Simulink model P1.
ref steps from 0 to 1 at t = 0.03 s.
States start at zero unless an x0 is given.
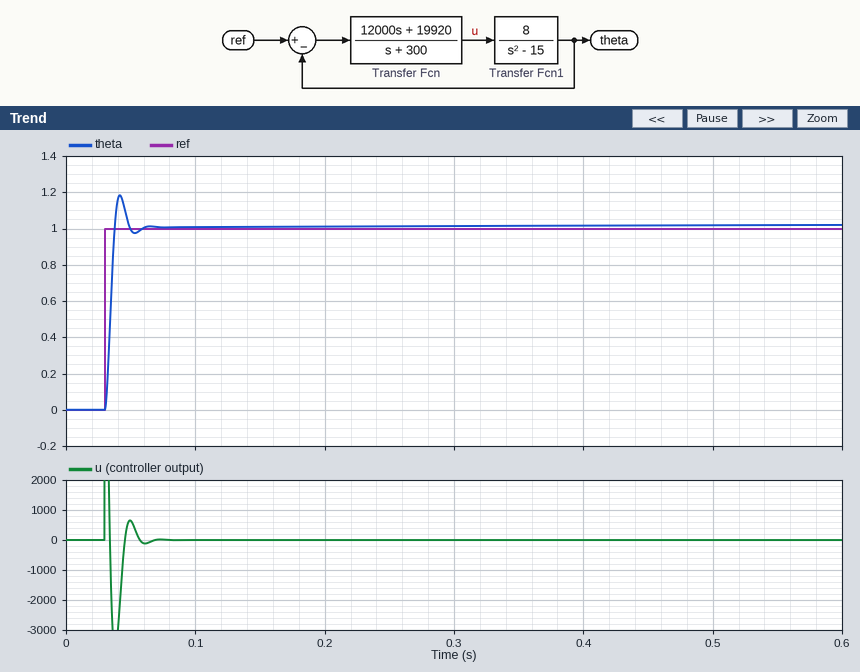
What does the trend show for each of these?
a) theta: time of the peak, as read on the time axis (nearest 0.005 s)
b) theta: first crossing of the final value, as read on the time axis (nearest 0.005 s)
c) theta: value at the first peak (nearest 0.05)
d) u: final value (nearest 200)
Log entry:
0.040 s
0.040 s
1.20
0
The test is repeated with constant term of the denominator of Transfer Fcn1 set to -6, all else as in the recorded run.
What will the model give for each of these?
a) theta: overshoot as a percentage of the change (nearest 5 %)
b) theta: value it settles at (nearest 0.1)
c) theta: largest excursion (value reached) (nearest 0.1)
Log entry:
15 %
1.0
1.2
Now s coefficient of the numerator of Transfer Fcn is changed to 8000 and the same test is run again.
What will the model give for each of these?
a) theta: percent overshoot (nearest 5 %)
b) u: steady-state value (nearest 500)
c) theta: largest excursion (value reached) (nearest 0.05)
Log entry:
10 %
0
1.10
